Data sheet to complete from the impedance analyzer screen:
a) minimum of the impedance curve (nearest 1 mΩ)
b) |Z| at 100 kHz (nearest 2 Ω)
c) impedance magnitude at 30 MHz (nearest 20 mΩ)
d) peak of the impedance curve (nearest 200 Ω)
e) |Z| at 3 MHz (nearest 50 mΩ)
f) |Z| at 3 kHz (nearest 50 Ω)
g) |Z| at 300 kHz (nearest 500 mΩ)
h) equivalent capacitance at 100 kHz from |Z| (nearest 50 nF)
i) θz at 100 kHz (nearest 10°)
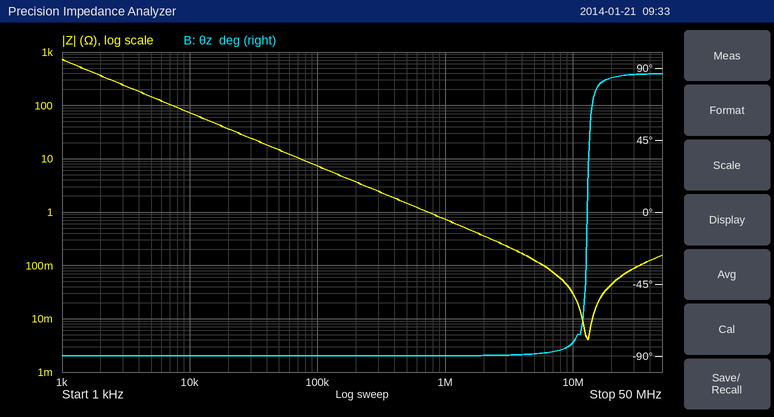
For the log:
4 mΩ
8 Ω
80 mΩ
800 Ω
250 mΩ
250 Ω
2.5 Ω
200 nF
-90°
